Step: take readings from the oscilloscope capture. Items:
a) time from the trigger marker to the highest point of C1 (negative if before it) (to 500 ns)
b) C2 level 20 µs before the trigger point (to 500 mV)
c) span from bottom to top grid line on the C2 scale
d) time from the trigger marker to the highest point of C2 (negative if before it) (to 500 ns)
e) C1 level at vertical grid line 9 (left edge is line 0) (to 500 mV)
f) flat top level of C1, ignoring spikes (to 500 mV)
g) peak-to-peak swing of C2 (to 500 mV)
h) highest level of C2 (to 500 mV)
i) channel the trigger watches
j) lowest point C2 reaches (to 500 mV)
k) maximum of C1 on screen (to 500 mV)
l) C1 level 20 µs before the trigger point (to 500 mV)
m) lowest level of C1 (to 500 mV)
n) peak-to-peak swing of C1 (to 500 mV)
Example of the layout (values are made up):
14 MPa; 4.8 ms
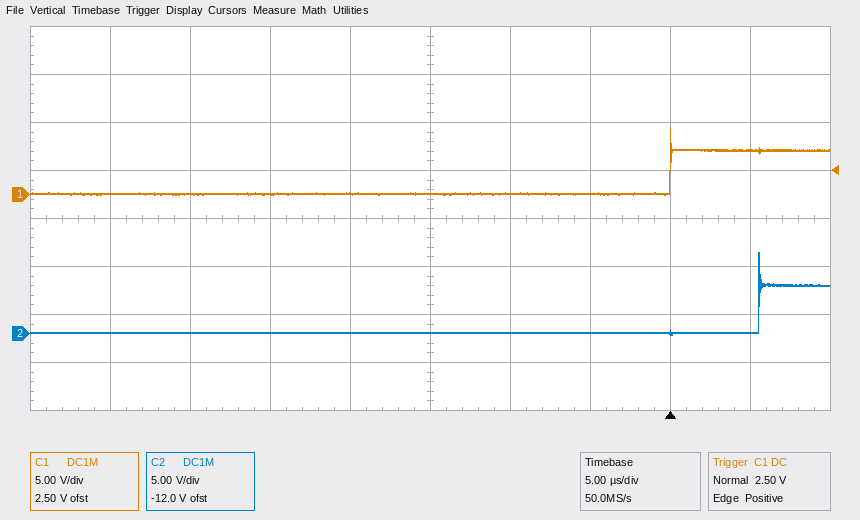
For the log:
0.0 µs; 0.0 V; 40 V; +5.5 µs; 4.5 V; 4.5 V; 8.5 V; 8.5 V; C1; 0.0 V; 7.0 V; 0.0 V; 0.0 V; 7.0 V
